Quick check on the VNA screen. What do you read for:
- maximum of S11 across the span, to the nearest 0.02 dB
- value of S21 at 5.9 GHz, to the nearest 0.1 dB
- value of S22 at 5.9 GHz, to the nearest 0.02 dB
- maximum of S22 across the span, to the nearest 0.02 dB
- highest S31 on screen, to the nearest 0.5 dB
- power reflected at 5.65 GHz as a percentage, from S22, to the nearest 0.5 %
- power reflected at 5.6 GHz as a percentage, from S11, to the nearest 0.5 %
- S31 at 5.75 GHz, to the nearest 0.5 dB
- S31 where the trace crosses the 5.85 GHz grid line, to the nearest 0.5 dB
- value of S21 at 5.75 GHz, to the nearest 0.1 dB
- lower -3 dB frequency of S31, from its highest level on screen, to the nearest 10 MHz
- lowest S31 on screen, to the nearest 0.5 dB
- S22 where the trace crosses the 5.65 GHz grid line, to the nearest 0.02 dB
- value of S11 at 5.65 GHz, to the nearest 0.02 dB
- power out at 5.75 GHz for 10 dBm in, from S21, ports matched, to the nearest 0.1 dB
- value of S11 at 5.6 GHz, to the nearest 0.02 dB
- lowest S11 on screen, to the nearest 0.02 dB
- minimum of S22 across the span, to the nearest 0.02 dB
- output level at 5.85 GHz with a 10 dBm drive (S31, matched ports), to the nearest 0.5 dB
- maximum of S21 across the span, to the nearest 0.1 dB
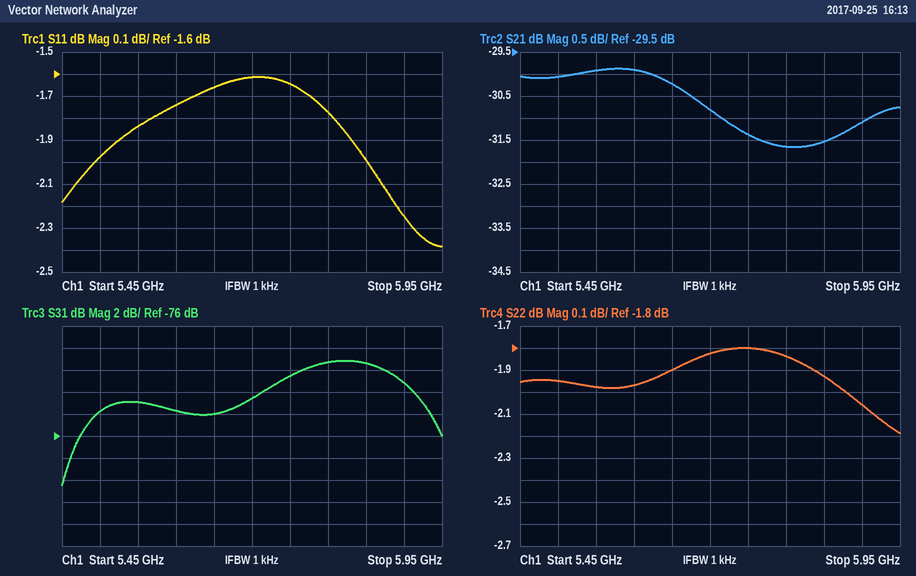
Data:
-1.62 dB
-31.1 dB
-2.06 dB
-1.80 dB
-69.0 dB
64.5 %
67.0 %
-70.5 dB
-69.5 dB
-31.4 dB
5.71 GHz
-80.5 dB
-1.90 dB
-1.66 dB
-21.4 dBm
-1.74 dB
-2.38 dB
-2.18 dB
-59.5 dBm
-29.9 dB
